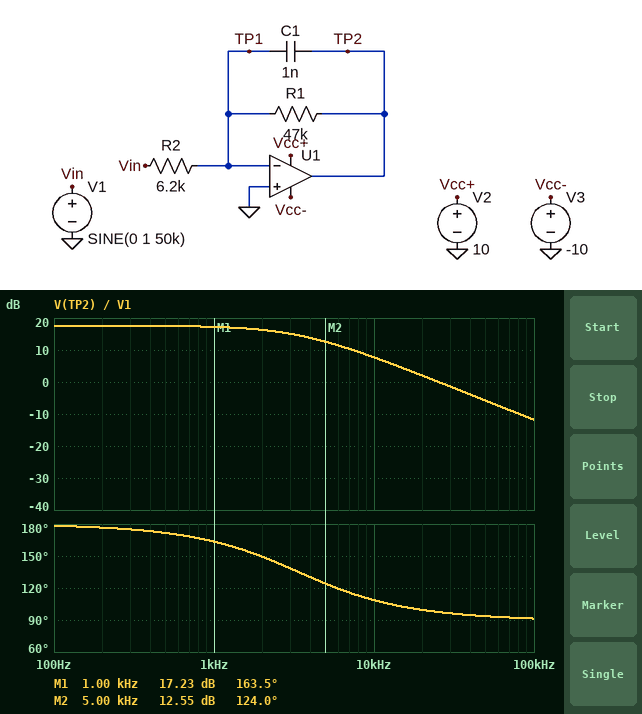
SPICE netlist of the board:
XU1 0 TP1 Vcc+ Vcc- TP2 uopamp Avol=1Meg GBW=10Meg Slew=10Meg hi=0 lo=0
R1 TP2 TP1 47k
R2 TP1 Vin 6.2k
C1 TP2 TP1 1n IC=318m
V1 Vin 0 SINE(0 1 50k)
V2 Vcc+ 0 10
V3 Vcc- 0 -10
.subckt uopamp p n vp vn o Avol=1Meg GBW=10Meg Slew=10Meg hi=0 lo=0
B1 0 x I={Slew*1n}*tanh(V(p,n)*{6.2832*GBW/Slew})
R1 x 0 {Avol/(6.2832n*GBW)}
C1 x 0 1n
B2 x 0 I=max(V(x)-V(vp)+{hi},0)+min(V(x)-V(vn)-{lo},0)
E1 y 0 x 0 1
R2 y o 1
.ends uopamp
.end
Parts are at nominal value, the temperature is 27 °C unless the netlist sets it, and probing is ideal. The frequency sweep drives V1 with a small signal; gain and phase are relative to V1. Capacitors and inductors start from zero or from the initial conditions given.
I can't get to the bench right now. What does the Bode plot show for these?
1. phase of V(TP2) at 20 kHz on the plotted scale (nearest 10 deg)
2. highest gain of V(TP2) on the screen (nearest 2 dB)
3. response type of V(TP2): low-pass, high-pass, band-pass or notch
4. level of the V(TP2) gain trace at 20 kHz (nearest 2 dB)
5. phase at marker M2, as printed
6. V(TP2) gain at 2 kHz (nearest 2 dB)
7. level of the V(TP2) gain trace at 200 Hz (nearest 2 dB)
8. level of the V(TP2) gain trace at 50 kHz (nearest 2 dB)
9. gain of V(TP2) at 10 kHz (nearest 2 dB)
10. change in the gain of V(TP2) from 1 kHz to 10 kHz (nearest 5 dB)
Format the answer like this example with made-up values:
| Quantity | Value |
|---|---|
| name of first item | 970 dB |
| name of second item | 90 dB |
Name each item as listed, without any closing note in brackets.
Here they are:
| Quantity | Value |
|---|---|
| phase of V(TP2) at 20 kHz on the plotted scale | 100 deg |
| highest gain of V(TP2) on the screen | 18 dB |
| response type of V(TP2): low-pass, high-pass, band-pass or notch | low-pass |
| level of the V(TP2) gain trace at 20 kHz | 2 dB |
| phase at marker M2, as printed | 124.0 deg |
| V(TP2) gain at 2 kHz | 16 dB |
| level of the V(TP2) gain trace at 200 Hz | 18 dB |
| level of the V(TP2) gain trace at 50 kHz | -6 dB |
| gain of V(TP2) at 10 kHz | 8 dB |
| change in the gain of V(TP2) from 1 kHz to 10 kHz | -10 dB |
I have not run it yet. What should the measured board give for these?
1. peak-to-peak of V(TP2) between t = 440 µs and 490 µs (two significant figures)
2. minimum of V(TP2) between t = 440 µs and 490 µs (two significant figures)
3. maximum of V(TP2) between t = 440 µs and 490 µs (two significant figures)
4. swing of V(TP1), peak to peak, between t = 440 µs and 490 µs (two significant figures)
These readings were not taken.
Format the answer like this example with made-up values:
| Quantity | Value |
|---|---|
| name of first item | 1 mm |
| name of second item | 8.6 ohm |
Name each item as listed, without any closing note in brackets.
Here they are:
| Quantity | Value |
|---|---|
| peak-to-peak of V(TP2) between t = 440 µs and 490 µs | 1.0 V |
| minimum of V(TP2) between t = 440 µs and 490 µs | -510 mV |
| maximum of V(TP2) between t = 440 µs and 490 µs | 510 mV |
| swing of V(TP1), peak to peak, between t = 440 µs and 490 µs | 5.1 mV |
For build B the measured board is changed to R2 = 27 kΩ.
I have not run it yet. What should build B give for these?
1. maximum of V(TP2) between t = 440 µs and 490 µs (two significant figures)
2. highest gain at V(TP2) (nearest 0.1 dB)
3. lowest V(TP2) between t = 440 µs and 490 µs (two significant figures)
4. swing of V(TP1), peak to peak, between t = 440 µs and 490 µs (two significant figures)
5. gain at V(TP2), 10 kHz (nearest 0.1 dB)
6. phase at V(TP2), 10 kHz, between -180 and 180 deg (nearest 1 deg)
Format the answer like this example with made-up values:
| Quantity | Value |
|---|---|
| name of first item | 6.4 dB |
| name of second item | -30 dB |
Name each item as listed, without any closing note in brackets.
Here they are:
| Quantity | Value |
|---|---|
| maximum of V(TP2) between t = 440 µs and 490 µs | 120 mV |
| highest gain at V(TP2) | 4.8 dB |
| lowest V(TP2) between t = 440 µs and 490 µs | -120 mV |
| swing of V(TP1), peak to peak, between t = 440 µs and 490 µs | 1.2 mV |
| gain at V(TP2), 10 kHz | -5.1 dB |
| phase at V(TP2), 10 kHz, between -180 and 180 deg | 109 deg |
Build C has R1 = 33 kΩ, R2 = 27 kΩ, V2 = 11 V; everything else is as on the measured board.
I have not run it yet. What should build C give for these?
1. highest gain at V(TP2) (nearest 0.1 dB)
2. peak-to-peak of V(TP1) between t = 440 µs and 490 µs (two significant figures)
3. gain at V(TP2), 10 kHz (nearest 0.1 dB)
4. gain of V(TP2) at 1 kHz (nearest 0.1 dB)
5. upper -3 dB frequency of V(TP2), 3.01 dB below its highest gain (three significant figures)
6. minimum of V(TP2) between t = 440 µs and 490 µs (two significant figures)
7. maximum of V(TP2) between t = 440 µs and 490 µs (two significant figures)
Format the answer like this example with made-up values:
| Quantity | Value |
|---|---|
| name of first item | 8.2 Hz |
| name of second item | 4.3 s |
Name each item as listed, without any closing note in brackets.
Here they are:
| Quantity | Value |
|---|---|
| highest gain at V(TP2) | 1.7 dB |
| peak-to-peak of V(TP1) between t = 440 µs and 490 µs | 1.2 mV |
| gain at V(TP2), 10 kHz | -5.5 dB |
| gain of V(TP2) at 1 kHz | 1.6 dB |
| upper -3 dB frequency of V(TP2), 3.01 dB below its highest gain | 4.82 kHz |
| minimum of V(TP2) between t = 440 µs and 490 µs | -120 mV |
| maximum of V(TP2) between t = 440 µs and 490 µs | 120 mV |
